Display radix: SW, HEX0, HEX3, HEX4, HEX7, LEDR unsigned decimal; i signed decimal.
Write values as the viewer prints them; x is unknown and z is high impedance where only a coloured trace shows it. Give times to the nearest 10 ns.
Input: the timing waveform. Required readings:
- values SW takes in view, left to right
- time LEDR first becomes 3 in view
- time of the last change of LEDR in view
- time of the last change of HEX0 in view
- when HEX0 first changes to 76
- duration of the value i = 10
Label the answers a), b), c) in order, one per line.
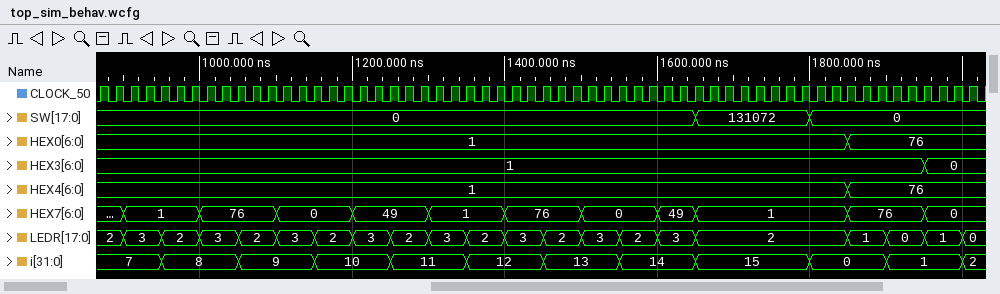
a) 0, 131072, 0
b) 900 ns
c) 2000 ns
d) 1850 ns
e) 1850 ns
f) 100 ns
